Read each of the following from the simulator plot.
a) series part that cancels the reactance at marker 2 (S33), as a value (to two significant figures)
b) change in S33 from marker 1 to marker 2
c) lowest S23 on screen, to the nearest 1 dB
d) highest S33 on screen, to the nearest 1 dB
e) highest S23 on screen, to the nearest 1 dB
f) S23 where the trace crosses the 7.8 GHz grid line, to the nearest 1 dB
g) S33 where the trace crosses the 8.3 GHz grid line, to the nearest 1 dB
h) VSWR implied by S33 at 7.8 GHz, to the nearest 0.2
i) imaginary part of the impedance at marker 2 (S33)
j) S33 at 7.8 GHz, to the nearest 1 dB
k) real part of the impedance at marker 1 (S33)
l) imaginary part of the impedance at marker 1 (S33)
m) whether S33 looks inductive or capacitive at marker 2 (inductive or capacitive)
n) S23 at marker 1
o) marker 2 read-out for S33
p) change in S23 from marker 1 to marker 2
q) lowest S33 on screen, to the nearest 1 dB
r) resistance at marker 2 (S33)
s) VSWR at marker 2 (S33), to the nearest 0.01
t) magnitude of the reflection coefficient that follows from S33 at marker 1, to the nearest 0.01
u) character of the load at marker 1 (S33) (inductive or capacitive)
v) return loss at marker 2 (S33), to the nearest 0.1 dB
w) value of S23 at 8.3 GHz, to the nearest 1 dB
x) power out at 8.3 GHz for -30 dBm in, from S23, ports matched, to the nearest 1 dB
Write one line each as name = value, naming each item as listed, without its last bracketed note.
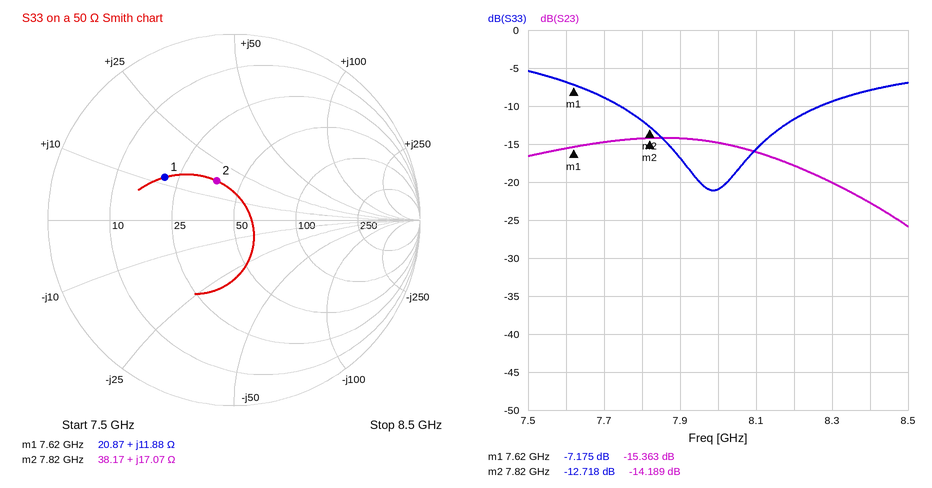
series part that cancels the reactance at marker 2 (S33), as a value = 1.2 pF
change in S33 from marker 1 to marker 2 = -5.543 dB
lowest S23 on screen, to the nearest 1 dB = -26 dB
highest S33 on screen, to the nearest 1 dB = -5 dB
highest S23 on screen, to the nearest 1 dB = -14 dB
S23 where the trace crosses the 7.8 GHz grid line, to the nearest 1 dB = -14 dB
S33 where the trace crosses the 8.3 GHz grid line, to the nearest 1 dB = -9 dB
VSWR implied by S33 at 7.8 GHz, to the nearest 0.2 = 1.6
imaginary part of the impedance at marker 2 = +17.07 Ω
S33 at 7.8 GHz, to the nearest 1 dB = -12 dB
real part of the impedance at marker 1 = 20.87 Ω
imaginary part of the impedance at marker 1 = +11.88 Ω
whether S33 looks inductive or capacitive at marker 2 = inductive
S23 at marker 1 = -15.363 dB
marker 2 read-out for S33 = -12.718 dB
change in S23 from marker 1 to marker 2 = 1.174 dB
lowest S33 on screen, to the nearest 1 dB = -21 dB
resistance at marker 2 = 38.17 Ω
VSWR at marker 2 (S33), to the nearest 0.01 = 1.60
magnitude of the reflection coefficient that follows from S33 at marker 1, to the nearest 0.01 = 0.44
character of the load at marker 1 (S33) = inductive
return loss at marker 2 (S33), to the nearest 0.1 dB = 12.7 dB
value of S23 at 8.3 GHz, to the nearest 1 dB = -20 dB
power out at 8.3 GHz for -30 dBm in, from S23, ports matched, to the nearest 1 dB = -50 dBm
